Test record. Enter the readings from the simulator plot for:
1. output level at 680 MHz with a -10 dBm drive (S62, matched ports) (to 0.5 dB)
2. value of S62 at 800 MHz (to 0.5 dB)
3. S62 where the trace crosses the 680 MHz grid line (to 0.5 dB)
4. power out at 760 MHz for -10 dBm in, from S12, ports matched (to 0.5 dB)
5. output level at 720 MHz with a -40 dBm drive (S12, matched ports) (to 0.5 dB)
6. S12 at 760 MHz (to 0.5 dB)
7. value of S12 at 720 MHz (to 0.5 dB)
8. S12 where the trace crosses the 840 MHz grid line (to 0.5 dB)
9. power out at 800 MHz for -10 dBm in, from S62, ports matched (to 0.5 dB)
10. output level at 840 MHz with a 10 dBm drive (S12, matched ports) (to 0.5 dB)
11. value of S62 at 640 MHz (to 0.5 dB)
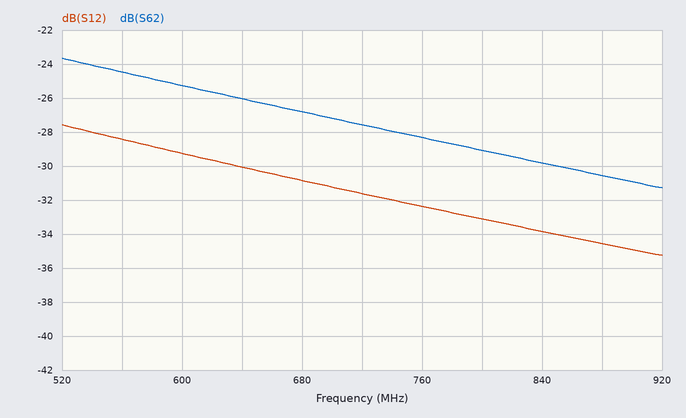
-37.0 dBm
-29.0 dB
-27.0 dB
-42.5 dBm
-71.5 dBm
-32.5 dB
-31.5 dB
-34.0 dB
-39.0 dBm
-24.0 dBm
-26.0 dB
